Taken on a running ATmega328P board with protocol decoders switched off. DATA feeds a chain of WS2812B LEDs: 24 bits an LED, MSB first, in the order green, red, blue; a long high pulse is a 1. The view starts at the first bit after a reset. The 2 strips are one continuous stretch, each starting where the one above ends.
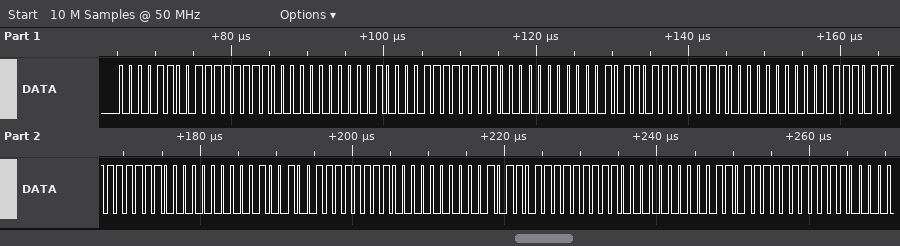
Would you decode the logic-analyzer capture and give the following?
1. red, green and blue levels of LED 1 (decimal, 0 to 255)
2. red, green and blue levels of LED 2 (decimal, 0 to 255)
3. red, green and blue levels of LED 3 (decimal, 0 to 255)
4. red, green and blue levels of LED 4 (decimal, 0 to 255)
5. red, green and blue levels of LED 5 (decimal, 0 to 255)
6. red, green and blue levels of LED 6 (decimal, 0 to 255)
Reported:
255, 12, 0
255, 16, 0
255, 22, 0
255, 29, 0
255, 36, 0
255, 45, 0
